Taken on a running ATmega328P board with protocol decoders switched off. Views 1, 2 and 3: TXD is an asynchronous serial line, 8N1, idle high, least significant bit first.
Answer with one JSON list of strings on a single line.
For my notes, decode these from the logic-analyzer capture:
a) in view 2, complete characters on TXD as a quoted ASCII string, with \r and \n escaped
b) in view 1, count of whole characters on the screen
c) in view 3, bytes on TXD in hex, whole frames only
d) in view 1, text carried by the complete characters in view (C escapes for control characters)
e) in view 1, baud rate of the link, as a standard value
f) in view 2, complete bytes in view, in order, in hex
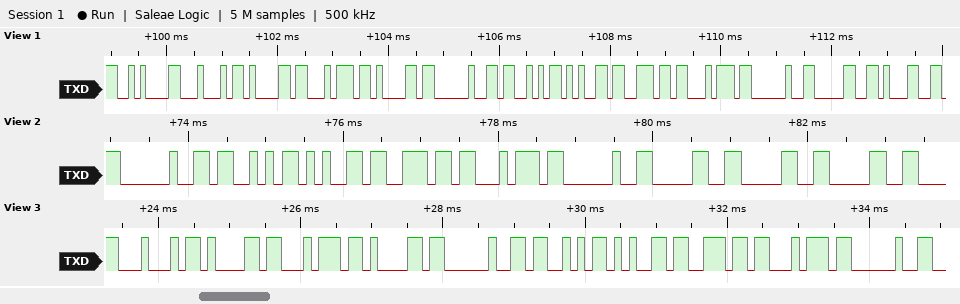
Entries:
["\" Sent 000\"", "13", "0x44 0x61 0x74 0x61 0x20 0x53 0x65 0x6E 0x74 0x20", "\"\\nData Sent 01\"", "9600 baud", "20 53 65 6E 74 20 30 30 30"]
